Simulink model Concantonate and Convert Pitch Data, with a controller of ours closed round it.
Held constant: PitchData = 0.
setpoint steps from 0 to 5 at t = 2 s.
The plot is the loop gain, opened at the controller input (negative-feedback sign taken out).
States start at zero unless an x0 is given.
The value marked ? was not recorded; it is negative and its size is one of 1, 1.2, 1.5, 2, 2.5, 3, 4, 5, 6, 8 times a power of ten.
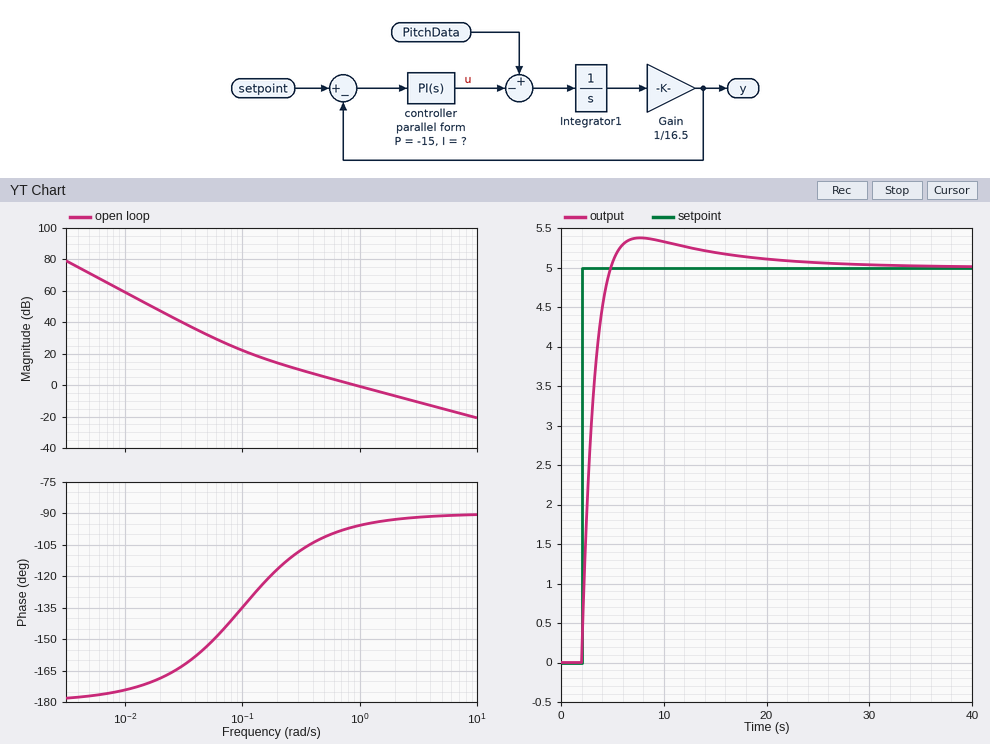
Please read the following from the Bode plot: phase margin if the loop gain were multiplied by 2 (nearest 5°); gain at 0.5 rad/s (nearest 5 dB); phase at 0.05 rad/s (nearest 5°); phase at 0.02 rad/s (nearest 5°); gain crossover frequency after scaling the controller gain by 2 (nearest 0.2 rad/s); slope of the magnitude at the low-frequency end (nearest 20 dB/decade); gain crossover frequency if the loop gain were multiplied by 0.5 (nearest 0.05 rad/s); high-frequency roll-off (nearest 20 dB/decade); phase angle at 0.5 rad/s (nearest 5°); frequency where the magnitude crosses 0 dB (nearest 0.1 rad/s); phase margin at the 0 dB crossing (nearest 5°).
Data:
85°
5 dB
-155°
-170°
1.8 rad/s
-40 dB/decade
0.45 rad/s
-20 dB/decade
-100°
0.9 rad/s
85°
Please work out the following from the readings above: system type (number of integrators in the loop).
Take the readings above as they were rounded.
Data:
2
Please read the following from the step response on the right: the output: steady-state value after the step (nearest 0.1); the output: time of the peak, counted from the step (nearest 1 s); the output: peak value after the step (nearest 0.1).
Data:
5.0
6 s
5.4
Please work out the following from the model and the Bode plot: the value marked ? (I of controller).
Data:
-1.5
